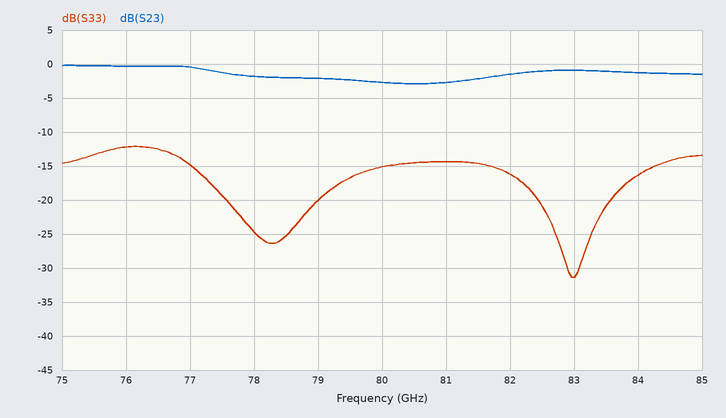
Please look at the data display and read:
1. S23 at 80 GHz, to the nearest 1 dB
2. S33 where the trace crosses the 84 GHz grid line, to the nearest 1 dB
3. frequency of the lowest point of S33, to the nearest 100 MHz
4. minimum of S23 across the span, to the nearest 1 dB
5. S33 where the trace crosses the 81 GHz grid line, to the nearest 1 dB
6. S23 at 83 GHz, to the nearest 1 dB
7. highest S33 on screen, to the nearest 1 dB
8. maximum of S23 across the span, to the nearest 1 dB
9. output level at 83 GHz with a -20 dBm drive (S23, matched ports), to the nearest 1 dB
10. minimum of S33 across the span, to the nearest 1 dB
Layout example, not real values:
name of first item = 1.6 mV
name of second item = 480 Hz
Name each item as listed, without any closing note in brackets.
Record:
S23 at 80 GHz, to the nearest 1 dB = -3 dB
S33 where the trace crosses the 84 GHz grid line, to the nearest 1 dB = -16 dB
frequency of the lowest point of S33, to the nearest 100 MHz = 83.0 GHz
minimum of S23 across the span, to the nearest 1 dB = -3 dB
S33 where the trace crosses the 81 GHz grid line, to the nearest 1 dB = -14 dB
S23 at 83 GHz, to the nearest 1 dB = -1 dB
highest S33 on screen, to the nearest 1 dB = -12 dB
maximum of S23 across the span, to the nearest 1 dB = 0 dB
output level at 83 GHz with a -20 dBm drive (S23, matched ports), to the nearest 1 dB = -21 dBm
minimum of S33 across the span, to the nearest 1 dB = -31 dB
